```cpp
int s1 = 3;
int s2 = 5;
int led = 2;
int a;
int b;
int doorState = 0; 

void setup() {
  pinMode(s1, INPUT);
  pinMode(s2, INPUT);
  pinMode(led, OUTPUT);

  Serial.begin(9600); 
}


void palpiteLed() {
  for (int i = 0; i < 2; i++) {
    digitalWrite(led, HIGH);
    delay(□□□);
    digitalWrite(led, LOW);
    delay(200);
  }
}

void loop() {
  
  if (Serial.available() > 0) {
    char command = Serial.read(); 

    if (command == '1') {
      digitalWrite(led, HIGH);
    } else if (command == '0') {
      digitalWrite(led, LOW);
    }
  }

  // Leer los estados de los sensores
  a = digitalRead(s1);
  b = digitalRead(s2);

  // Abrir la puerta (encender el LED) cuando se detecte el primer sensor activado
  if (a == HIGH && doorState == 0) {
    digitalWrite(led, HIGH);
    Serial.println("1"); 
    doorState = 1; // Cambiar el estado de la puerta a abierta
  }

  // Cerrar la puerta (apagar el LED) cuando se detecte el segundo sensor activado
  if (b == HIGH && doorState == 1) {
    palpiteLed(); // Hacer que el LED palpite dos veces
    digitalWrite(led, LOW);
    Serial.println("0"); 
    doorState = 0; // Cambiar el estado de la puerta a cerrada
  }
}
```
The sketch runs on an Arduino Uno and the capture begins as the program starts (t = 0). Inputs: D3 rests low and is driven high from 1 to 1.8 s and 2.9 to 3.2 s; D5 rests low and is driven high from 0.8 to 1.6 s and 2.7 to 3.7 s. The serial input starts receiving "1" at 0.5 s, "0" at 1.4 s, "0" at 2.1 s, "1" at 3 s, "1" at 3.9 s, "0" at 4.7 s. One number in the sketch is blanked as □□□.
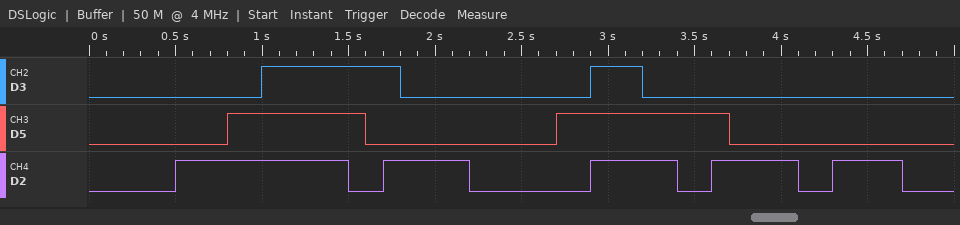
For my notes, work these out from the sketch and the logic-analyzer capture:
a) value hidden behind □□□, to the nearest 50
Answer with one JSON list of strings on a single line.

["500"]
